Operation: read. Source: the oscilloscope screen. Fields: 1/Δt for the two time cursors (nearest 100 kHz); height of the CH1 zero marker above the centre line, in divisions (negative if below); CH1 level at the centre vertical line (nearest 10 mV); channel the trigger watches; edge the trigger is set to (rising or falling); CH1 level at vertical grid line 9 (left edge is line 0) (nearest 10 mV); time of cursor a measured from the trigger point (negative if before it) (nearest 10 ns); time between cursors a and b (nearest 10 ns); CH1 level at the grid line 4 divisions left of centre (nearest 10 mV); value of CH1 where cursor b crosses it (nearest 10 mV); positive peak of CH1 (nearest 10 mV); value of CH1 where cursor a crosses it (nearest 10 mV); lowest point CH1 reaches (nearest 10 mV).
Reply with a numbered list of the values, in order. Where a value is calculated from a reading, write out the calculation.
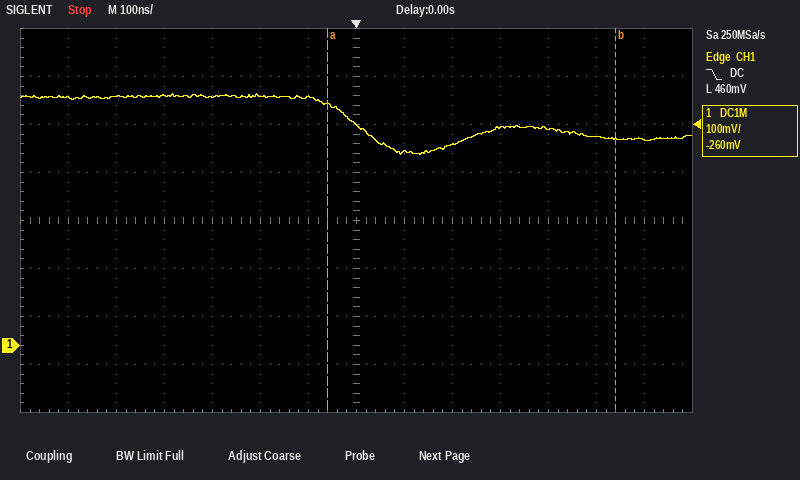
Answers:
1. 1 / 600 ns ≈ 1.7 MHz
2. -2.6 div
3. 460 mV
4. CH1
5. falling
6. 420 mV
7. -60 ns
8. 600 ns
9. 520 mV
10. 430 mV
11. 520 mV
12. 500 mV
13. 400 mV
